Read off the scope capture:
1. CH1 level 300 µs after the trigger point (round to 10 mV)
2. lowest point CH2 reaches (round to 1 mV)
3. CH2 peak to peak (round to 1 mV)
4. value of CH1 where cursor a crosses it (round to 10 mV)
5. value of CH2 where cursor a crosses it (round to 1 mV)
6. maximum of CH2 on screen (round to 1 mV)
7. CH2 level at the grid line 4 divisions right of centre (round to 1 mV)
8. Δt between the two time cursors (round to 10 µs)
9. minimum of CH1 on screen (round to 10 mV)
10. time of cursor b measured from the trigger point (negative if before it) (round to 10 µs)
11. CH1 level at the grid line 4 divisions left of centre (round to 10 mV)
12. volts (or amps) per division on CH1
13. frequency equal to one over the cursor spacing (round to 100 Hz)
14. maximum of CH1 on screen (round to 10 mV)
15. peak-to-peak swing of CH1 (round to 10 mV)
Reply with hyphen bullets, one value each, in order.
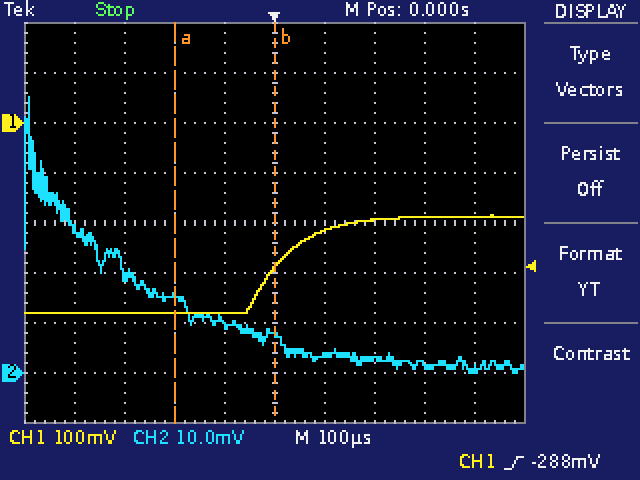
- -190 mV
- 0 mV
- 55 mV
- -380 mV
- 15 mV
- 55 mV
- 1 mV
- 200 µs
- -380 mV
- 0 µs
- -380 mV
- 100 mV
- 5.0 kHz
- -180 mV
- 200 mV
